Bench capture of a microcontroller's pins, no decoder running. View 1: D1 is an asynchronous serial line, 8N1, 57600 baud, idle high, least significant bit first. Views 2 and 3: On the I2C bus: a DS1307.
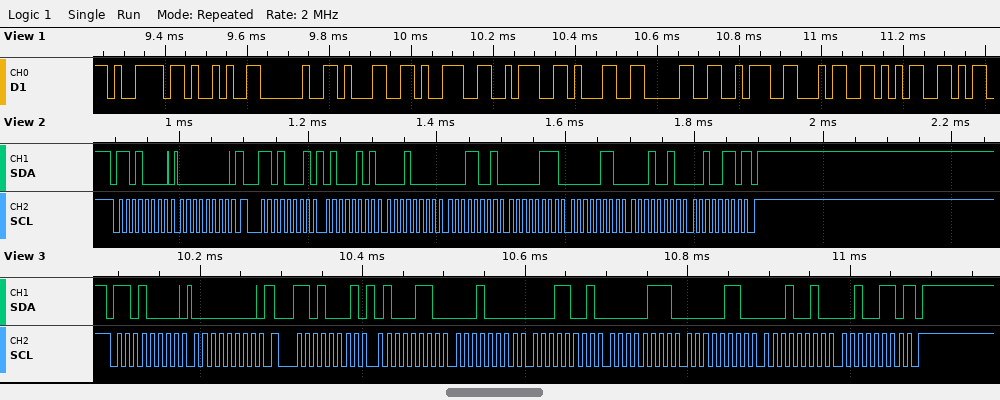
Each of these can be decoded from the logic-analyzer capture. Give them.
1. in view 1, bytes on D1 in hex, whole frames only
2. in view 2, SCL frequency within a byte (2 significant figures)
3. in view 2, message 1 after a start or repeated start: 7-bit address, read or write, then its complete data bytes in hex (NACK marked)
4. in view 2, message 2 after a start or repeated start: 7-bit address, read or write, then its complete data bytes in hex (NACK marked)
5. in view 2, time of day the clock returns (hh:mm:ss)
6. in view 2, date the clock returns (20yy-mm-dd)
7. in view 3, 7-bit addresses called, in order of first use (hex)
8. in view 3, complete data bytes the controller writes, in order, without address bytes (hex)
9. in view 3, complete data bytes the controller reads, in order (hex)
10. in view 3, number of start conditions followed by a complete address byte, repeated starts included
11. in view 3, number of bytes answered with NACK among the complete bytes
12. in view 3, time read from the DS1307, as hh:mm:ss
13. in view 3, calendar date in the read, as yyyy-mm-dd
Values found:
79 29 20 31 39 3A 31 30 3A 34 35
100 kHz
0x68 write: 00
0x68 read: 45 10 19 07 06 12 26 NACK
19:10:45
2026-12-06
0x68
00
46 10 19 07 06 12 26
2
1
19:10:46
2026-12-06
